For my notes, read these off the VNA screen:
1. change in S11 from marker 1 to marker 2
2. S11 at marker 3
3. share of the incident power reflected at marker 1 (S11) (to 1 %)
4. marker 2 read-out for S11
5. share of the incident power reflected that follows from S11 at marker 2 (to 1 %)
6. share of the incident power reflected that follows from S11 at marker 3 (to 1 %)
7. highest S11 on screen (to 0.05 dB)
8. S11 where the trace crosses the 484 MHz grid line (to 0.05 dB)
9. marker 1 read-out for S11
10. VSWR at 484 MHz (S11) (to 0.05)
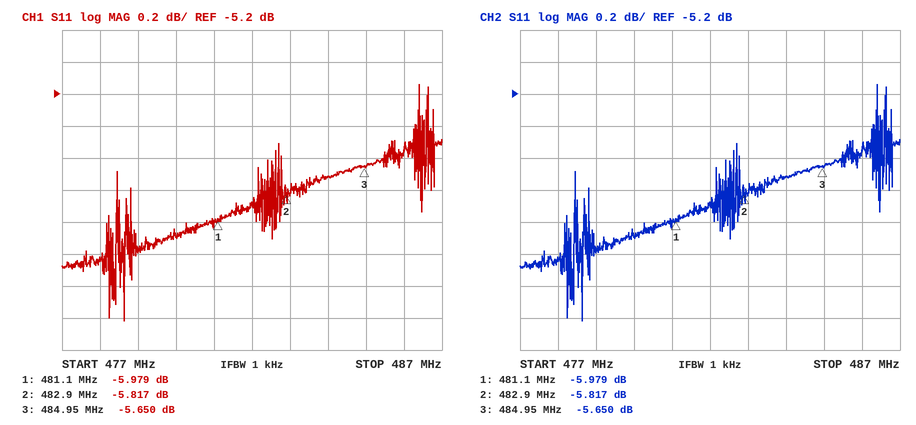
0.162 dB
-5.650 dB
25 %
-5.817 dB
26 %
27 %
-5.15 dB
-5.70 dB
-5.979 dB
3.15
